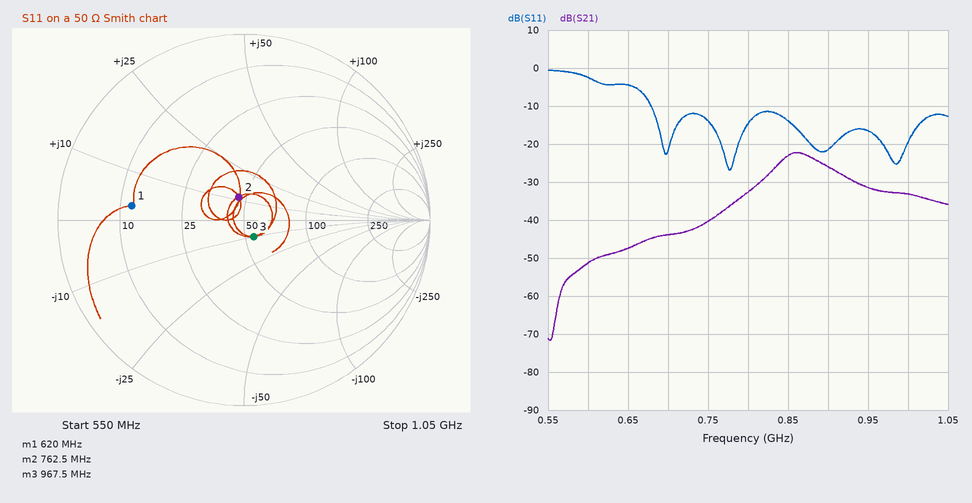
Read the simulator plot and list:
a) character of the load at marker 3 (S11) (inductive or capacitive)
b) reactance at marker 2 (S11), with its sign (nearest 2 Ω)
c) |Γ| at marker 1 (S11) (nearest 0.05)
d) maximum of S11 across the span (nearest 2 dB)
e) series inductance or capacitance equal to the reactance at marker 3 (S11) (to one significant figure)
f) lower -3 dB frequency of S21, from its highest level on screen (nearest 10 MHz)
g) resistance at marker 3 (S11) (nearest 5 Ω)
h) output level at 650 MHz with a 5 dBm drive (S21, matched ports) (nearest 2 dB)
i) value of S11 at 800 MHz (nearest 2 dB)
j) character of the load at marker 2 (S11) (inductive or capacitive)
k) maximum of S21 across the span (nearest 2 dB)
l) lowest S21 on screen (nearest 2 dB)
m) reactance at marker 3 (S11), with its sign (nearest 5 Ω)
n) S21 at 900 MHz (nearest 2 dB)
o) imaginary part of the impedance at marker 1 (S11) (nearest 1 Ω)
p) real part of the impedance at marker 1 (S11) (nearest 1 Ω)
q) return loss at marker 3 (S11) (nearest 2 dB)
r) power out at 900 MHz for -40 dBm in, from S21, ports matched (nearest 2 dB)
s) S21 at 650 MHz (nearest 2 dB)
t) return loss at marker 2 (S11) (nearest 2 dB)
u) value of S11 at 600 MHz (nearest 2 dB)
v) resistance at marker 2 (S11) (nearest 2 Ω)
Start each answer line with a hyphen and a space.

- capacitive
- +12 Ω
- 0.60
- 0 dB
- 20 pF
- 840 MHz
- 55 Ω
- -42 dBm
- -14 dB
- inductive
- -22 dB
- -72 dB
- -10 Ω
- -26 dB
- +3 Ω
- 12 Ω
- 20 dB
- -66 dBm
- -48 dB
- 18 dB
- -2 dB
- 46 Ω
